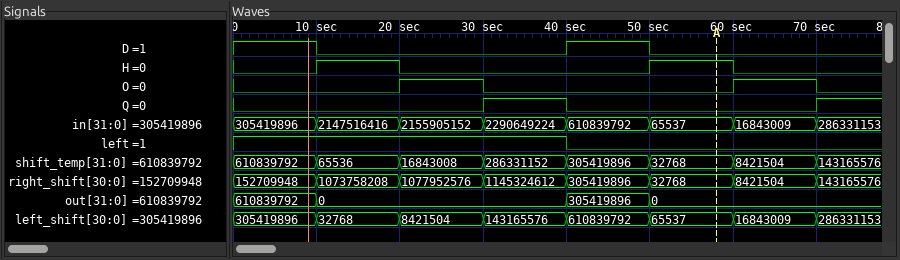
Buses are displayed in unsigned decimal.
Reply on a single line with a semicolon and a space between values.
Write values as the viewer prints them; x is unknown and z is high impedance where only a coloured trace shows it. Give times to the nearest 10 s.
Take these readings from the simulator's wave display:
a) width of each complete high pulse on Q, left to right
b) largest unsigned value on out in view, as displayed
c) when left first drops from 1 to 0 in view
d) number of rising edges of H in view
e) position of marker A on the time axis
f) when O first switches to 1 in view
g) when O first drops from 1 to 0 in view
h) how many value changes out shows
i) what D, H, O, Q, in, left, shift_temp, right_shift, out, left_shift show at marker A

10 s; 610839792; 40 s; 2; 60 s; 20 s; 30 s; 3; D=0, H=1, O=0, Q=0, in=65537, left=0, shift_temp=32768, right_shift=32768, out=0, left_shift=65537
